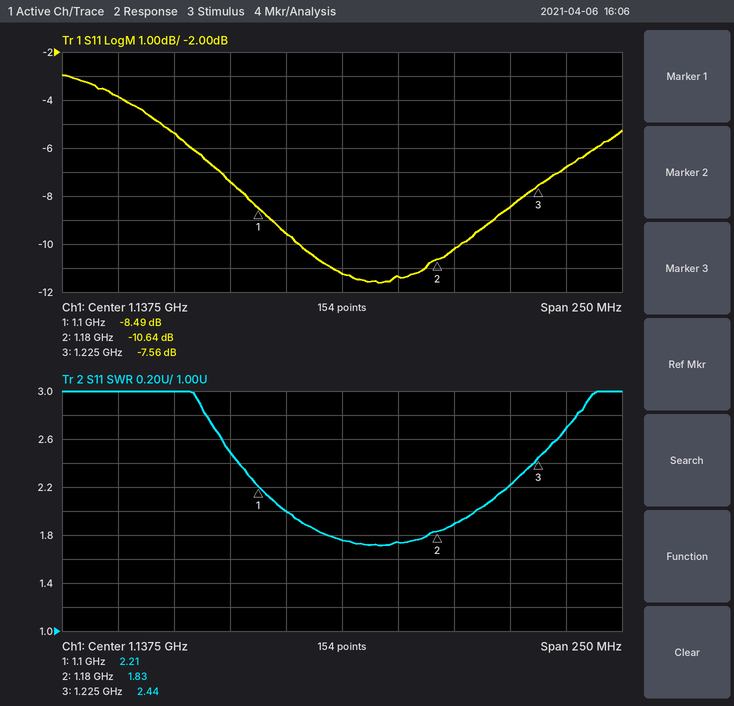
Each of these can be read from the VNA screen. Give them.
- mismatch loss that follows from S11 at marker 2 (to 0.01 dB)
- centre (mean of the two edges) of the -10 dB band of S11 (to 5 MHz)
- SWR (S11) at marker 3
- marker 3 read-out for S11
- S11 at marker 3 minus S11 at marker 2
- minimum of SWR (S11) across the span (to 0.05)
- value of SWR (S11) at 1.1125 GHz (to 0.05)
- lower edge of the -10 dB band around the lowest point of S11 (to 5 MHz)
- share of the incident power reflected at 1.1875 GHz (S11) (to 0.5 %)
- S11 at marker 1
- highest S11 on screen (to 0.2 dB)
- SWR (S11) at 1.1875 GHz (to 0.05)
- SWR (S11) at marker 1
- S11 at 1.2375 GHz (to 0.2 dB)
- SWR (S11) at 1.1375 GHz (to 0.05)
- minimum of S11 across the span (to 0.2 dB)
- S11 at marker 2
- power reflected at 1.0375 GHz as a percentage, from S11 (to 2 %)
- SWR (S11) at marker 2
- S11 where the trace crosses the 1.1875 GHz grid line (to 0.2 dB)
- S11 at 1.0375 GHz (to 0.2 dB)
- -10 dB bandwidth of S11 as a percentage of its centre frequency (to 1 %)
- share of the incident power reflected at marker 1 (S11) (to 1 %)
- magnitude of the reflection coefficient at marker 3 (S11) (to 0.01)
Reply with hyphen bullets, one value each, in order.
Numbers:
- 0.39 dB
- 1.155 GHz
- 2.44
- -7.56 dB
- 3.08 dB
- 1.70
- 2.00
- 1.120 GHz
- 9.5 %
- -8.49 dB
- -3.0 dB
- 1.90
- 2.21
- -6.8 dB
- 1.75
- -11.6 dB
- -10.64 dB
- 42 %
- 1.83
- -10.2 dB
- -3.8 dB
- 6 %
- 14 %
- 0.42
